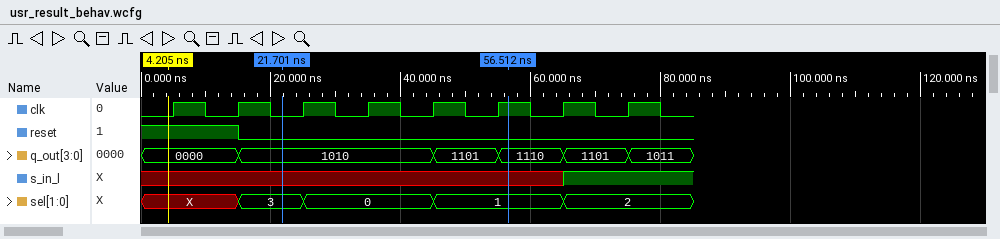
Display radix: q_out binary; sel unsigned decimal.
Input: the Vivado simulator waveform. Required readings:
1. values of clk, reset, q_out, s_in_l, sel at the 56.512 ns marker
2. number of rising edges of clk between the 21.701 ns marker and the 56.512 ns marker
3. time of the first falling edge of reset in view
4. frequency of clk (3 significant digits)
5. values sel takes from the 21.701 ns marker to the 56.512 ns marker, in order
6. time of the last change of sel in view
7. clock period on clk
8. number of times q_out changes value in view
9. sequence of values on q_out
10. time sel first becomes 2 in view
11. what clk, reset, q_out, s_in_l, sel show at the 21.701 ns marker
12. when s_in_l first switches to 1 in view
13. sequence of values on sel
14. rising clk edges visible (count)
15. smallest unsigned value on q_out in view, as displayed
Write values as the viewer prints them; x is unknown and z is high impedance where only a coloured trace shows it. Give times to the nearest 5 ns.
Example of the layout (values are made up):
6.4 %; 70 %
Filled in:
clk=1, reset=0, q_out=1110, s_in_l=x, sel=1; 4; 15 ns; 100 MHz; 3, 0, 1; 65 ns; 10 ns; 5; 0000, 1010, 1101, 1110, 1101, 1011; 65 ns; clk=0, reset=0, q_out=1010, s_in_l=x, sel=3; 65 ns; X, 3, 0, 1, 2; 8; 0000
